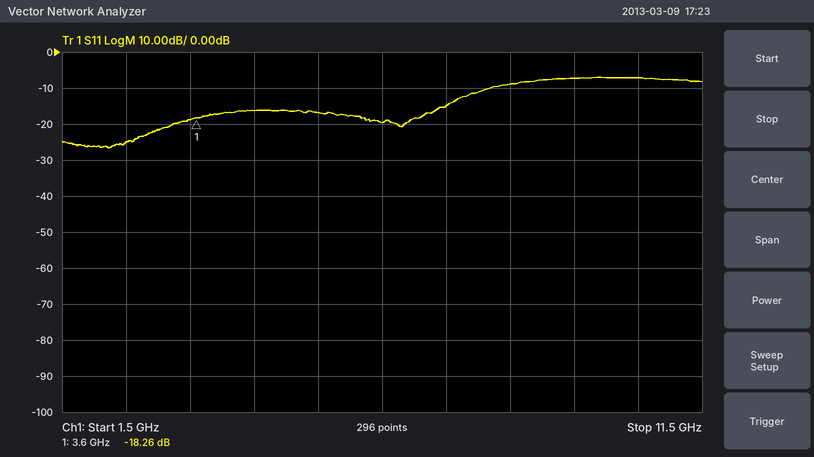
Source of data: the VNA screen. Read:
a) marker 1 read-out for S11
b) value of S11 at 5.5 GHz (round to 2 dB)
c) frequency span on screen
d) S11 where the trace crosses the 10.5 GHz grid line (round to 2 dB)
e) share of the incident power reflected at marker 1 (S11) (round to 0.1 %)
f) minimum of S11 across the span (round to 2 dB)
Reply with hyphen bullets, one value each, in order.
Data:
- -18.26 dB
- -16 dB
- 10 GHz
- -8 dB
- 1.5 %
- -26 dB
